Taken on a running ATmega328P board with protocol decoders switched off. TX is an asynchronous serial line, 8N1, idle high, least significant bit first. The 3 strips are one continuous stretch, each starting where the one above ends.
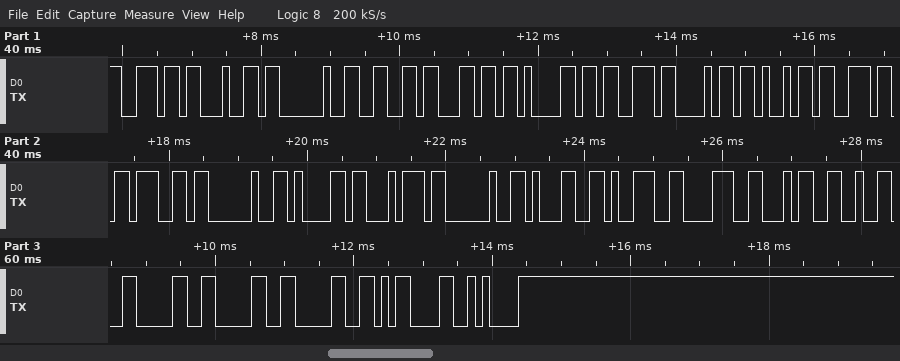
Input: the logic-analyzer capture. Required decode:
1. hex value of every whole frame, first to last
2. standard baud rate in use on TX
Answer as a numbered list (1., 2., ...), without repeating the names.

1. 6E 64 20 66 6C 61 73 68 69 6E 67 20 61 74 20 31 39 38 34 32 30 30 30 0D 0A
2. 9600 baud
